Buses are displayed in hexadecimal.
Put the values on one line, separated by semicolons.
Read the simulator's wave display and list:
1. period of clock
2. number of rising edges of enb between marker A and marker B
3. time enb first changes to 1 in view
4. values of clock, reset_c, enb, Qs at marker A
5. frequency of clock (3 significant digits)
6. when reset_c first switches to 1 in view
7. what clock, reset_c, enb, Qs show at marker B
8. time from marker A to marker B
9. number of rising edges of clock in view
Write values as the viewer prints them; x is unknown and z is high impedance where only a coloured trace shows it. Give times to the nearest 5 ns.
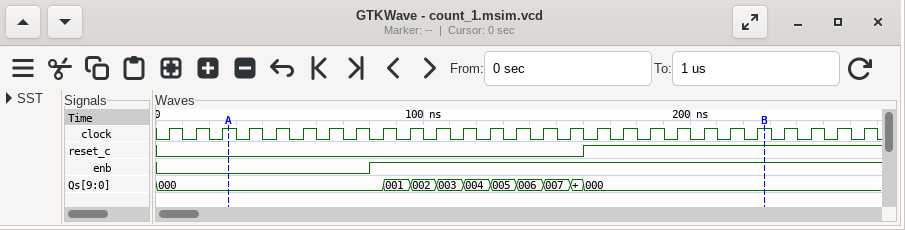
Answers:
10 ns; 1; 80 ns; clock=1, reset_c=0, enb=0, Qs=000; 100 MHz; 160 ns; clock=1, reset_c=1, enb=1, Qs=000; 200 ns; 27
